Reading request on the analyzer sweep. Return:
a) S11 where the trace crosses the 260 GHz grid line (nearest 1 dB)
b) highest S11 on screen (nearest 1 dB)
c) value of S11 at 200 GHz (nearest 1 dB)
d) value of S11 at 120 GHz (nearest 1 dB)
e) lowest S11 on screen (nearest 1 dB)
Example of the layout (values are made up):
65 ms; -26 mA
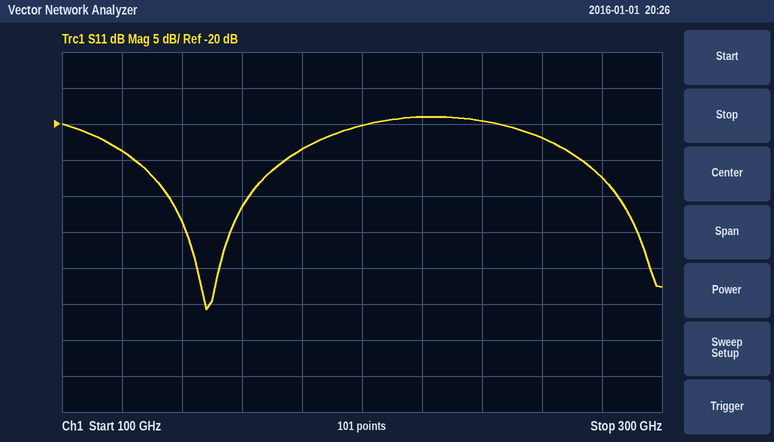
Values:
-22 dB; -19 dB; -20 dB; -24 dB; -46 dB
